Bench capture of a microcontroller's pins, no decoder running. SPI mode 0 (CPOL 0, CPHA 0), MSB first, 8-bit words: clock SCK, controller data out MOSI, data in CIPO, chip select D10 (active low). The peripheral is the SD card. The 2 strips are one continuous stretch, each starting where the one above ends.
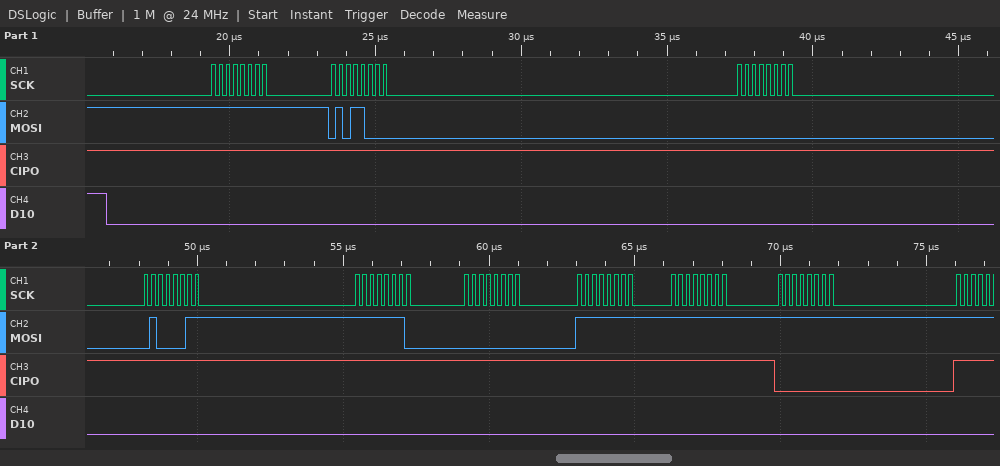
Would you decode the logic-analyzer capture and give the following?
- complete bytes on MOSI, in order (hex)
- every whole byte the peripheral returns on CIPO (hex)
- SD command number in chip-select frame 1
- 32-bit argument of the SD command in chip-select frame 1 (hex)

FF 58 00 43 FE 00 FF FF FF
FF FF FF FF FF FF FF FF 00
CMD24
0x0043FE00
